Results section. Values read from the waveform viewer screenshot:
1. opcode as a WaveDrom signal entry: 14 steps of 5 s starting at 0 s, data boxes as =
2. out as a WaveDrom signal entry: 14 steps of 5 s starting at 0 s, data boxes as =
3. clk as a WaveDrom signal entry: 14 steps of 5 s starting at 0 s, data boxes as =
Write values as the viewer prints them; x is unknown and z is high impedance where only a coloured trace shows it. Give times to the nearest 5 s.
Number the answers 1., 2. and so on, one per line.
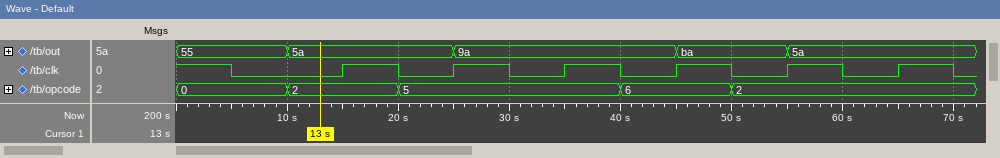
1. {name: 'opcode', wave: '=.=.=...=.=...', data: '0 2 5 6 2'}
2. {name: 'out', wave: '=.=..=...=.=..', data: '55 5a 9a ba 5a'}
3. {name: 'clk', wave: '10.10101010101'}
